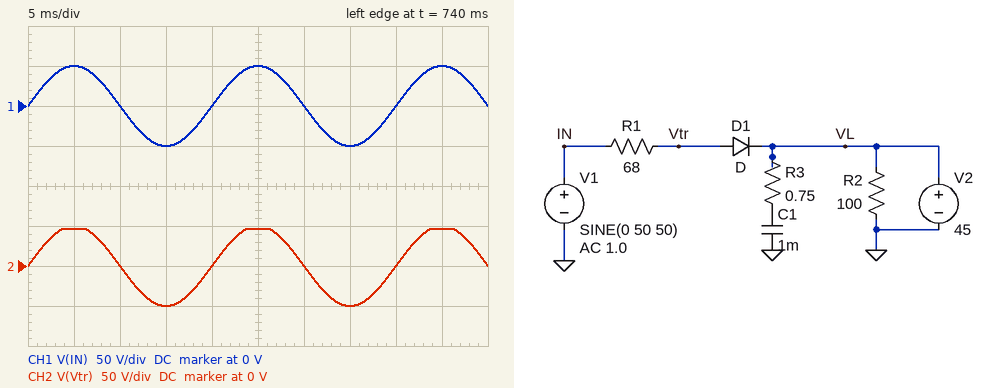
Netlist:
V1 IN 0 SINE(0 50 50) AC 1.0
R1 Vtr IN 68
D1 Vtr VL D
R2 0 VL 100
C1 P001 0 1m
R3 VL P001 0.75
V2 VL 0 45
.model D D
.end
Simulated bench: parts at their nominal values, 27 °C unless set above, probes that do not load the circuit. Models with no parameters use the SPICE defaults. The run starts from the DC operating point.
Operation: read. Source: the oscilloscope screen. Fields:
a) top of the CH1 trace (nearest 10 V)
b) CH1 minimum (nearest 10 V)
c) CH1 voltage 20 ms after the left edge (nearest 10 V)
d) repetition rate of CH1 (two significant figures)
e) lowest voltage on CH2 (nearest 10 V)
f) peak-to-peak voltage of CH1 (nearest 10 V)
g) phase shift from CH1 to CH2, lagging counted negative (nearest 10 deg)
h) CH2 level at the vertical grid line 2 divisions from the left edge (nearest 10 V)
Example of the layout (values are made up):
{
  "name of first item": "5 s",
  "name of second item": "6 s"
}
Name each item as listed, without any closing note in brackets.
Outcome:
{
  "top of the CH1 trace": "50 V",
  "CH1 minimum": "-50 V",
  "CH1 voltage 20 ms after the left edge": "0 V",
  "repetition rate of CH1": "50 Hz",
  "lowest voltage on CH2": "-50 V",
  "peak-to-peak voltage of CH1": "100 V",
  "phase shift from CH1 to CH2, lagging counted negative": "0 deg",
  "CH2 level at the vertical grid line 2 divisions from the left edge": "0 V"
}
